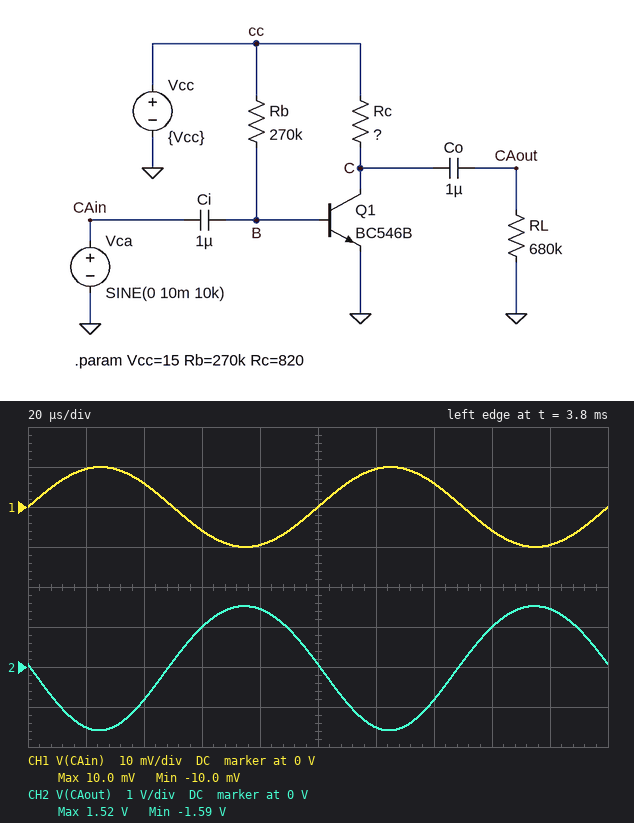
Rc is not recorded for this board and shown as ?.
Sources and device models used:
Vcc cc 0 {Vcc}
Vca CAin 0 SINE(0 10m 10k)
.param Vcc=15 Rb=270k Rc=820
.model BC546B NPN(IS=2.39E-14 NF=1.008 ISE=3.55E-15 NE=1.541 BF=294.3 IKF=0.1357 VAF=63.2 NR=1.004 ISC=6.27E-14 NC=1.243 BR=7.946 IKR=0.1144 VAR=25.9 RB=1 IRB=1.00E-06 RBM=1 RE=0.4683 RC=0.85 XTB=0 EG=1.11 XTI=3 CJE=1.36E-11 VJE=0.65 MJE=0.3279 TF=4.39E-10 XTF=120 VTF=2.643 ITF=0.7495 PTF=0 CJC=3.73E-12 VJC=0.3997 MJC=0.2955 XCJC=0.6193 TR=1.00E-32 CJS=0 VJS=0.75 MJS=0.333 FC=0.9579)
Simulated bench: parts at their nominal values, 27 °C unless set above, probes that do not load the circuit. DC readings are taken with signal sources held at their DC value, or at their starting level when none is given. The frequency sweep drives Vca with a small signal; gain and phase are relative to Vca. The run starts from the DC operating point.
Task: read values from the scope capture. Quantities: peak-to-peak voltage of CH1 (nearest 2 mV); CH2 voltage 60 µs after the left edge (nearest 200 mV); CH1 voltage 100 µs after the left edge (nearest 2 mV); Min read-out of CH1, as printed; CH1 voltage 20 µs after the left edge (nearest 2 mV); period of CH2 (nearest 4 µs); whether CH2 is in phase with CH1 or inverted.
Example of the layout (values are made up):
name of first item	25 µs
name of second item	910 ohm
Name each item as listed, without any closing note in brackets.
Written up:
peak-to-peak voltage of CH1	20 mV
CH2 voltage 60 µs after the left edge	1.0 V
CH1 voltage 100 µs after the left edge	0 V
Min read-out of CH1, as printed	-10.0 mV
CH1 voltage 20 µs after the left edge	10 mV
period of CH2	100 µs
whether CH2 is in phase with CH1 or inverted	inverted
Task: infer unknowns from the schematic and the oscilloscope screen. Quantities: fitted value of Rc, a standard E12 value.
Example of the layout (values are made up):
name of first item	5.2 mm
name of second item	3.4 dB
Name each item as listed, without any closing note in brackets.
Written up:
fitted value of Rc, a standard E12 value	390 Ω
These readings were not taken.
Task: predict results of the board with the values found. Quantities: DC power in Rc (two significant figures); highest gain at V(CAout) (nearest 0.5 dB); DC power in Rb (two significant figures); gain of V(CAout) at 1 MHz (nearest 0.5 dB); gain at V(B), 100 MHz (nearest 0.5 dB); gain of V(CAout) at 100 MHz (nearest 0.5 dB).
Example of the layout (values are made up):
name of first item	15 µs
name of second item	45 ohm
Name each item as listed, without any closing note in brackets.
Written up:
DC power in Rc	94 mW
highest gain at V(CAout)	44.0 dB
DC power in Rb	760 µW
gain of V(CAout) at 1 MHz	44.0 dB
gain at V(B), 100 MHz	0 dB
gain of V(CAout) at 100 MHz	43.0 dB
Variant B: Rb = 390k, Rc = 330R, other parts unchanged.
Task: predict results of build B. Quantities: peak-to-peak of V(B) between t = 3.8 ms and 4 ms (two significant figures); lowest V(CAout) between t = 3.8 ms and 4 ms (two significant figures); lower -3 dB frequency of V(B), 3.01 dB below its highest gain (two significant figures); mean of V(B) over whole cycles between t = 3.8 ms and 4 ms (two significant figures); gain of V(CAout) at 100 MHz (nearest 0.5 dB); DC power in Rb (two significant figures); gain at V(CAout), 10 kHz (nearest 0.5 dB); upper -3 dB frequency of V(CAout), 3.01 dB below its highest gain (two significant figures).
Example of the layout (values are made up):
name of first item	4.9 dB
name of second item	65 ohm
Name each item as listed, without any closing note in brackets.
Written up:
peak-to-peak of V(B) between t = 3.8 ms and 4 ms	20 mV
lowest V(CAout) between t = 3.8 ms and 4 ms	-1.1 V
lower -3 dB frequency of V(B), 3.01 dB below its highest gain	190 Hz
mean of V(B) over whole cycles between t = 3.8 ms and 4 ms	700 mV
gain of V(CAout) at 100 MHz	40.0 dB
DC power in Rb	520 µW
gain at V(CAout), 10 kHz	40.5 dB
upper -3 dB frequency of V(CAout), 3.01 dB below its highest gain	230 MHz
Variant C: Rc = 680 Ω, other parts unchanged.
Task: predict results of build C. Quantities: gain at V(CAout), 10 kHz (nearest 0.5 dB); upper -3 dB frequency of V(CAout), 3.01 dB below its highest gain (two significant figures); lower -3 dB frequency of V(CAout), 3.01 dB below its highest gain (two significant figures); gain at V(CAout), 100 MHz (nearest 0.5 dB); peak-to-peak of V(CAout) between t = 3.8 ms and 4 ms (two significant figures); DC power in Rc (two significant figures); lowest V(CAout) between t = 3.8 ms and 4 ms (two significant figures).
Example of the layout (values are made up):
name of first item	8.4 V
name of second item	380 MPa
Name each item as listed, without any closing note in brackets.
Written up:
gain at V(CAout), 10 kHz	48.0 dB
upper -3 dB frequency of V(CAout), 3.01 dB below its highest gain	110 MHz
lower -3 dB frequency of V(CAout), 3.01 dB below its highest gain	270 Hz
gain at V(CAout), 100 MHz	45.0 dB
peak-to-peak of V(CAout) between t = 3.8 ms and 4 ms	4.9 V
DC power in Rc	150 mW
lowest V(CAout) between t = 3.8 ms and 4 ms	-2.5 V
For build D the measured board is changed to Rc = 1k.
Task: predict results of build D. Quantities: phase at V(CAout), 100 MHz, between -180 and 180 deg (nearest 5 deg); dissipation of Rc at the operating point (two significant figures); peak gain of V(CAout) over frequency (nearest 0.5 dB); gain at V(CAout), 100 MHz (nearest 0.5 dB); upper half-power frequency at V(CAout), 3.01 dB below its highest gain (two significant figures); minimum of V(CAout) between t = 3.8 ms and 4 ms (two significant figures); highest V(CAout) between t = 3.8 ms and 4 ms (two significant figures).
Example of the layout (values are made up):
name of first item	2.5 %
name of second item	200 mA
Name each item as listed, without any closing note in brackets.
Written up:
phase at V(CAout), 100 MHz, between -180 and 180 deg	105 deg
dissipation of Rc at the operating point	190 mW
peak gain of V(CAout) over frequency	50.5 dB
gain at V(CAout), 100 MHz	43.5 dB
upper half-power frequency at V(CAout), 3.01 dB below its highest gain	50 MHz
minimum of V(CAout) between t = 3.8 ms and 4 ms	-1.1 V
highest V(CAout) between t = 3.8 ms and 4 ms	4.6 V
